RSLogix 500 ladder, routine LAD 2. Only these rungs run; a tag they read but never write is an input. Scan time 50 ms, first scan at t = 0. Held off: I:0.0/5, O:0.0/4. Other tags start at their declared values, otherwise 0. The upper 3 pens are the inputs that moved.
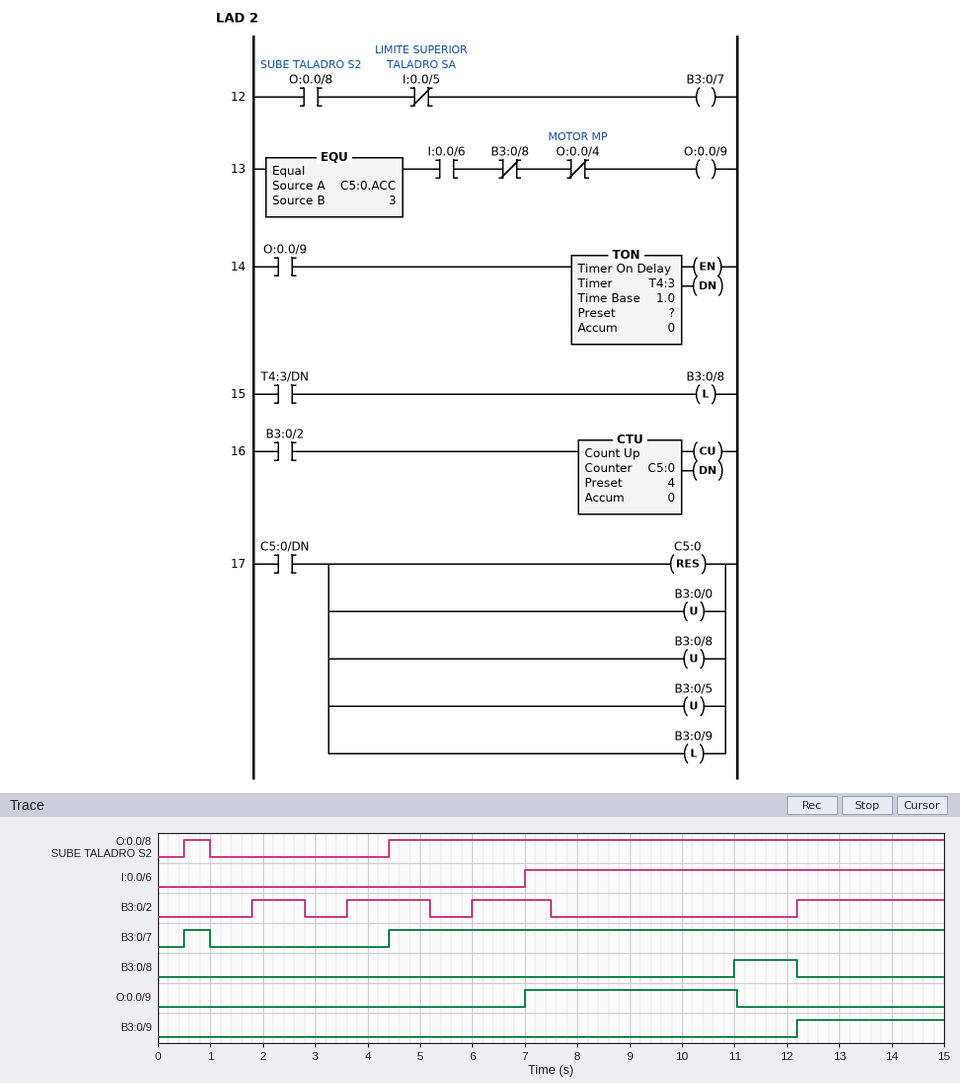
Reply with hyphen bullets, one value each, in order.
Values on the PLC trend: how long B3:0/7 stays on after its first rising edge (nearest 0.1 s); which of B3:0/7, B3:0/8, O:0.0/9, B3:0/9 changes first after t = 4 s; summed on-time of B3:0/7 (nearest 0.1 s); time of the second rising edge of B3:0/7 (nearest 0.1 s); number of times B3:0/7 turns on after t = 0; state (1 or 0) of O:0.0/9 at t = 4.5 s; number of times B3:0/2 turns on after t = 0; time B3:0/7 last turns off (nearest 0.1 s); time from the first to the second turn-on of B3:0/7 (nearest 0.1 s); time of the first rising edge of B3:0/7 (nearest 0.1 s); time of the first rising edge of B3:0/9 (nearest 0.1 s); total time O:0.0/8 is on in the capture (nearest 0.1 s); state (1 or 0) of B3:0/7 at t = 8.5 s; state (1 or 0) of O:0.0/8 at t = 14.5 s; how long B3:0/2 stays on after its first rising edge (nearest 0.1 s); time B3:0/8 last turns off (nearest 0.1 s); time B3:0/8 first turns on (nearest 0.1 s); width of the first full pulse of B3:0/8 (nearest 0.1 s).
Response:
- 0.5 s
- B3:0/7
- 11.1 s
- 4.4 s
- 2
- 0
- 4
- 1.0 s
- 3.9 s
- 0.5 s
- 12.2 s
- 11.1 s
- 1
- 1
- 1.0 s
- 12.2 s
- 11.0 s
- 1.2 s
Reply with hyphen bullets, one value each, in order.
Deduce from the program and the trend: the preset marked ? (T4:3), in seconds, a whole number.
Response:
- 4 s
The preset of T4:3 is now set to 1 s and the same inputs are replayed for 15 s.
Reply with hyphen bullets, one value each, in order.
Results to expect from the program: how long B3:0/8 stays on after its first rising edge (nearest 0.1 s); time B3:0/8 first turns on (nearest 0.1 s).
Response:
- 4.2 s
- 8.0 s
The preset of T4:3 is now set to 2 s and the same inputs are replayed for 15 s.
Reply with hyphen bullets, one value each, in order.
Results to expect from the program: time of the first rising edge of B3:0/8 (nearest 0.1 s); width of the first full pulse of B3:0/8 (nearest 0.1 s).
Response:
- 9.0 s
- 3.2 s
